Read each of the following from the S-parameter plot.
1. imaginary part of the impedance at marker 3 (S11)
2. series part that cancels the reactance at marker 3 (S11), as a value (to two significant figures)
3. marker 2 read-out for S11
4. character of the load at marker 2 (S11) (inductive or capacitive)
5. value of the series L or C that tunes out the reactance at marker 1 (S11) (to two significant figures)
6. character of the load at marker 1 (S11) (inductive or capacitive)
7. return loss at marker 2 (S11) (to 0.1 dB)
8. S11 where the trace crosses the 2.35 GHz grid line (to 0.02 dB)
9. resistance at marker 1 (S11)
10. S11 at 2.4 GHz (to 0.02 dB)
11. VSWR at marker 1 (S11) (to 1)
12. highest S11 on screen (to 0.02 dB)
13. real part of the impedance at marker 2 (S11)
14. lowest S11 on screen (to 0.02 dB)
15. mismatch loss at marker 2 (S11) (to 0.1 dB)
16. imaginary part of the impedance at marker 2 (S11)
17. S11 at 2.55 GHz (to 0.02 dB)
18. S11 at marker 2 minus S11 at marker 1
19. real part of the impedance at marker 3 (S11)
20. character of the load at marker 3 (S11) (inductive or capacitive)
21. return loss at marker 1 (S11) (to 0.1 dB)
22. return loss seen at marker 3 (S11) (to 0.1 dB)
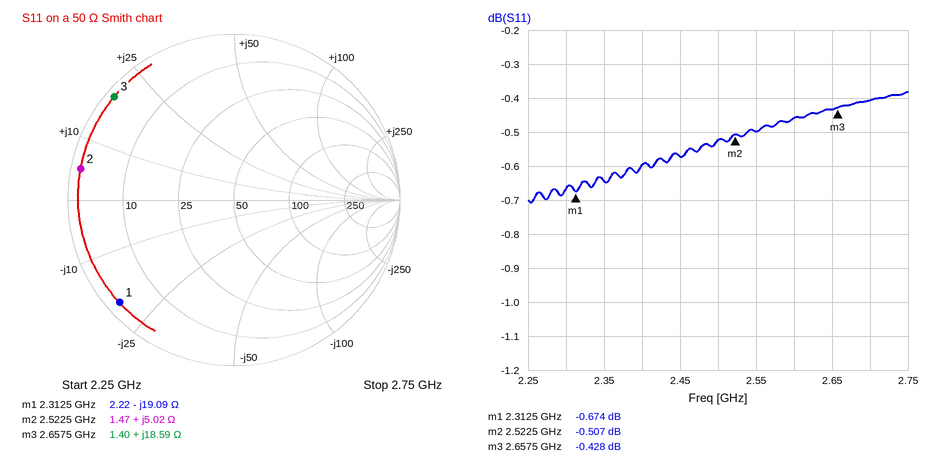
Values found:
+18.59 Ω
3.2 pF
-0.507 dB
inductive
1.3 nH
capacitive
0.5 dB
-0.64 dB
2.22 Ω
-0.60 dB
26
-0.38 dB
1.47 Ω
-0.70 dB
9.6 dB
+5.02 Ω
-0.50 dB
0.167 dB
1.40 Ω
inductive
0.7 dB
0.4 dB
